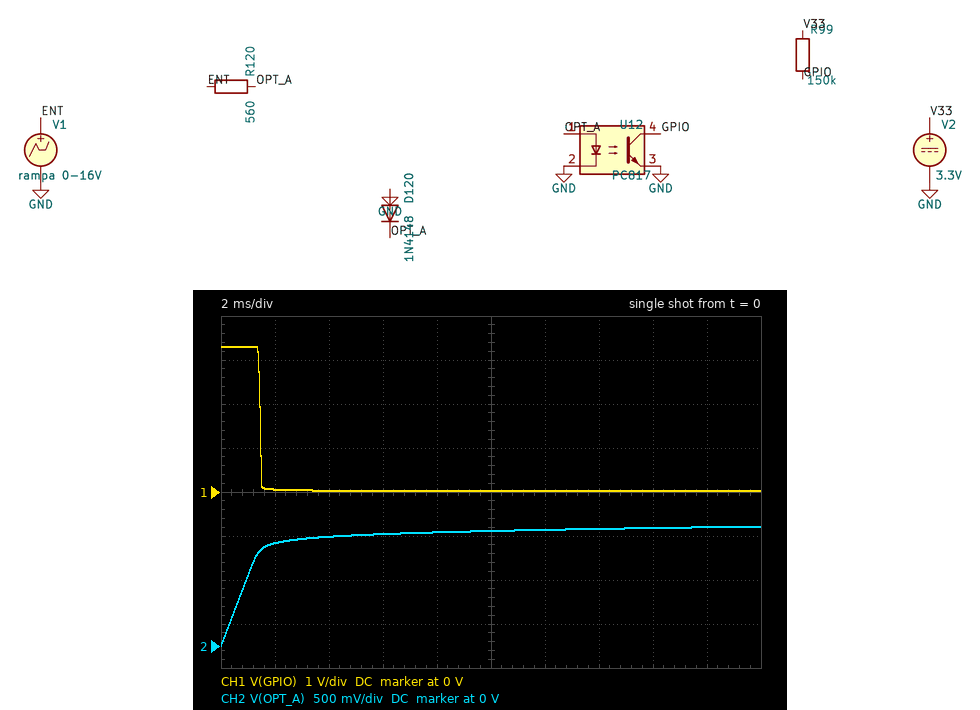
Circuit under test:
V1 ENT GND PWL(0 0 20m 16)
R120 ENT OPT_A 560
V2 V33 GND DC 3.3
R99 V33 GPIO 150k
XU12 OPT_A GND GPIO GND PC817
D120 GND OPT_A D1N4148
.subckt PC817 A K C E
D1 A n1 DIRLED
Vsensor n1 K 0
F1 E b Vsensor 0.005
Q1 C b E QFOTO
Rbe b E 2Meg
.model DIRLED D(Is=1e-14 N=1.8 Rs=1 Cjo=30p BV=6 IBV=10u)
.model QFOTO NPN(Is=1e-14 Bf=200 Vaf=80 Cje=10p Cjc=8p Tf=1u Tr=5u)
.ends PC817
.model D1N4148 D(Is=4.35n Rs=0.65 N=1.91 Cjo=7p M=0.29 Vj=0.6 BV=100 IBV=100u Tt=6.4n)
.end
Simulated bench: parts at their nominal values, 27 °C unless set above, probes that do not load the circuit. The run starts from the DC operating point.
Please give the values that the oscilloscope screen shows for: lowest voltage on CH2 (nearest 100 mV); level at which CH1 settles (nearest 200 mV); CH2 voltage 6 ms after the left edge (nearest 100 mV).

0 V
0 V
1.3 V
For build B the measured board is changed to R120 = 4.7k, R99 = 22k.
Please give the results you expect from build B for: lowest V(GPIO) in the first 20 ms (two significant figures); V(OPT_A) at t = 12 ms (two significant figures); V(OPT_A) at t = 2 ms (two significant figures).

65 mV
1.2 V
1.1 V
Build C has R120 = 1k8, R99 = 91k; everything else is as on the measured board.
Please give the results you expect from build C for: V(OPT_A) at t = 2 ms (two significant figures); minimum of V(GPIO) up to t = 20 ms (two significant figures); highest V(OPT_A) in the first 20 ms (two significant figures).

1.1 V
28 mV
1.3 V
